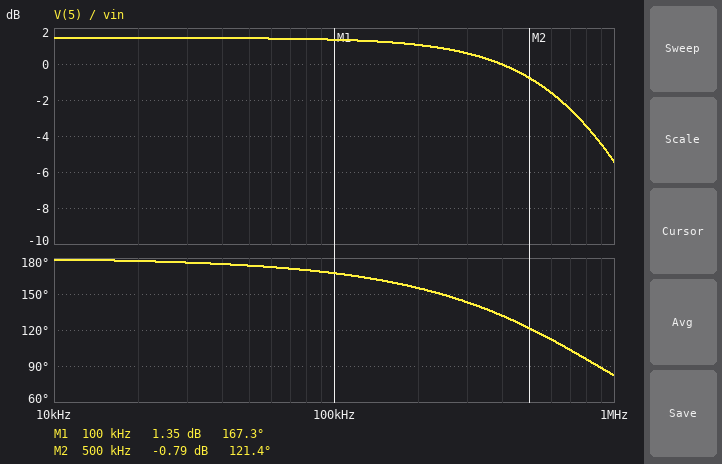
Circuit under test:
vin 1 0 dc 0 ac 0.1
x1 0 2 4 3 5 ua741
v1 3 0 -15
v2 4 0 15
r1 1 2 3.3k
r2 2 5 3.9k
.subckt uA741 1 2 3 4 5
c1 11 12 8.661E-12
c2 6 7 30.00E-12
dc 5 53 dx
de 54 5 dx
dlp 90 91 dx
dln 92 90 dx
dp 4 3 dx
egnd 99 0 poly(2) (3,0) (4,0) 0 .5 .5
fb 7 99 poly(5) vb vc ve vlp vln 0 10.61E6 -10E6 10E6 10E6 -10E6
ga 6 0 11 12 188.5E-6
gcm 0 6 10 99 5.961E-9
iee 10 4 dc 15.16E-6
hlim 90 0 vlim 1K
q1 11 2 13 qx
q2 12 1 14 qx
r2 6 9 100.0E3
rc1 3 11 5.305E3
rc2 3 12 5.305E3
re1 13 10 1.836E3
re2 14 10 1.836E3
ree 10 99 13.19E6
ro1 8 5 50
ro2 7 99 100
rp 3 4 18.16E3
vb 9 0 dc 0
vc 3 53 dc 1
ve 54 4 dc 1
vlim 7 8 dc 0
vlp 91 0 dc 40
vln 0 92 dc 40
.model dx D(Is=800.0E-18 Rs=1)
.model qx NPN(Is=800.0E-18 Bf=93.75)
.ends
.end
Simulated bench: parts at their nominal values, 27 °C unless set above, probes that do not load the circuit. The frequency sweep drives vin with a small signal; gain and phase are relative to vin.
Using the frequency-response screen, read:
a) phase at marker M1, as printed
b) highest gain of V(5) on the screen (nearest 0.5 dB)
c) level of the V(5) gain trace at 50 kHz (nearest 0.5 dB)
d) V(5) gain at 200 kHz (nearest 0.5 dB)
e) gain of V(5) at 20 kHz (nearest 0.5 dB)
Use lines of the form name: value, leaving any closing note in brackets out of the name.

phase at marker M1, as printed: 167.3 deg
highest gain of V(5) on the screen: 1.5 dB
level of the V(5) gain trace at 50 kHz: 1.5 dB
V(5) gain at 200 kHz: 1.0 dB
gain of V(5) at 20 kHz: 1.5 dB
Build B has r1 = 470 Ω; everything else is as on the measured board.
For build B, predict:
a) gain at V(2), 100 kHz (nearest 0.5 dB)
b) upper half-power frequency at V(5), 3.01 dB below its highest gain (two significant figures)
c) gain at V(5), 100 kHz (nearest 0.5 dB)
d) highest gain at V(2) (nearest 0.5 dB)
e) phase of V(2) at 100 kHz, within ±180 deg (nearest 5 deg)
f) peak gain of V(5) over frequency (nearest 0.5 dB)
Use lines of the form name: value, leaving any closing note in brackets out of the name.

gain at V(2), 100 kHz: -4.0 dB
upper half-power frequency at V(5), 3.01 dB below its highest gain: 110 kHz
gain at V(5), 100 kHz: 16.0 dB
highest gain at V(2): -0.5 dB
phase of V(2) at 100 kHz, within ±180 deg: 50 deg
peak gain of V(5) over frequency: 18.5 dB
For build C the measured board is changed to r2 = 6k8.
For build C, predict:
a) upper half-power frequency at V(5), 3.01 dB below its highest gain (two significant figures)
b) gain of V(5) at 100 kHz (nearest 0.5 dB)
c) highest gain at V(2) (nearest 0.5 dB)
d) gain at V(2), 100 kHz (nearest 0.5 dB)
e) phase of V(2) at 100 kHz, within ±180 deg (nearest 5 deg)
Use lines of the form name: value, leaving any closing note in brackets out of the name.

upper half-power frequency at V(5), 3.01 dB below its highest gain: 390 kHz
gain of V(5) at 100 kHz: 6.0 dB
highest gain at V(2): -2.5 dB
gain at V(2), 100 kHz: -14.0 dB
phase of V(2) at 100 kHz, within ±180 deg: 75 deg
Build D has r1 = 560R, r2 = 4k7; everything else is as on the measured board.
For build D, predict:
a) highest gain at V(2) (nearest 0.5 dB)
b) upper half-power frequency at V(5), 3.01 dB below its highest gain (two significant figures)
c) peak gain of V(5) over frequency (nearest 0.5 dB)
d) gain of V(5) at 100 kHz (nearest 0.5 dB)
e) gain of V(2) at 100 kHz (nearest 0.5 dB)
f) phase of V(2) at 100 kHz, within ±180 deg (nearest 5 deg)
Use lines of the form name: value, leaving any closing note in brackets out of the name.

highest gain at V(2): -0.5 dB
upper half-power frequency at V(5), 3.01 dB below its highest gain: 110 kHz
peak gain of V(5) over frequency: 18.5 dB
gain of V(5) at 100 kHz: 16.0 dB
gain of V(2) at 100 kHz: -4.0 dB
phase of V(2) at 100 kHz, within ±180 deg: 50 deg
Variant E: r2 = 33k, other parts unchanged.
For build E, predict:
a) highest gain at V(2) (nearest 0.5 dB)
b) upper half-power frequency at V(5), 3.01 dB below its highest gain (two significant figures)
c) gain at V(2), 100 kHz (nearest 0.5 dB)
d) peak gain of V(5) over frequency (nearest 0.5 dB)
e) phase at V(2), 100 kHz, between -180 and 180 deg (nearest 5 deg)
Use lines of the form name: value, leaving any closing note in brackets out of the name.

highest gain at V(2): -0.5 dB
upper half-power frequency at V(5), 3.01 dB below its highest gain: 95 kHz
gain at V(2), 100 kHz: -3.0 dB
peak gain of V(5) over frequency: 20.0 dB
phase at V(2), 100 kHz, between -180 and 180 deg: 45 deg
